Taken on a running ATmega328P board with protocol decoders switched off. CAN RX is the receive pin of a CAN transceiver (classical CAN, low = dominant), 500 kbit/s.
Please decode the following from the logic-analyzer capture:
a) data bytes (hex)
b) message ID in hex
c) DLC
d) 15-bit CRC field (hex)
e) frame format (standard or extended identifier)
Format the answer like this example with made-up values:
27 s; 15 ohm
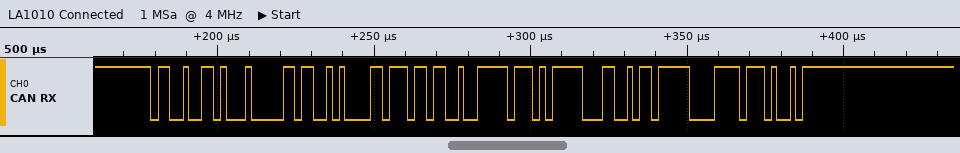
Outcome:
2C A1 BB 64 FF 5F 32 DF; 0x64D; 8; 0x0F74; standard
